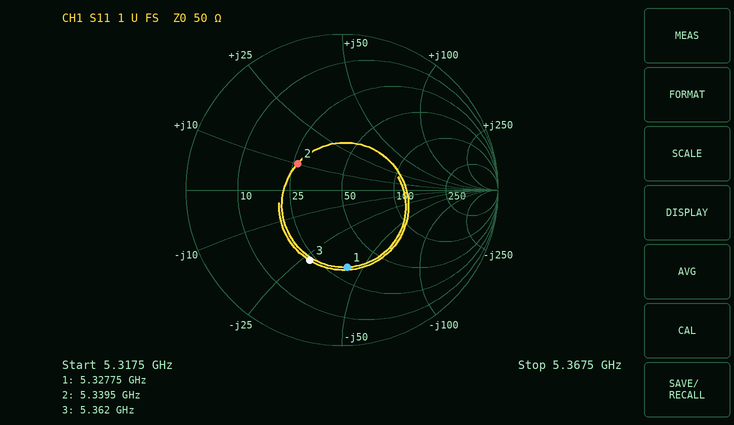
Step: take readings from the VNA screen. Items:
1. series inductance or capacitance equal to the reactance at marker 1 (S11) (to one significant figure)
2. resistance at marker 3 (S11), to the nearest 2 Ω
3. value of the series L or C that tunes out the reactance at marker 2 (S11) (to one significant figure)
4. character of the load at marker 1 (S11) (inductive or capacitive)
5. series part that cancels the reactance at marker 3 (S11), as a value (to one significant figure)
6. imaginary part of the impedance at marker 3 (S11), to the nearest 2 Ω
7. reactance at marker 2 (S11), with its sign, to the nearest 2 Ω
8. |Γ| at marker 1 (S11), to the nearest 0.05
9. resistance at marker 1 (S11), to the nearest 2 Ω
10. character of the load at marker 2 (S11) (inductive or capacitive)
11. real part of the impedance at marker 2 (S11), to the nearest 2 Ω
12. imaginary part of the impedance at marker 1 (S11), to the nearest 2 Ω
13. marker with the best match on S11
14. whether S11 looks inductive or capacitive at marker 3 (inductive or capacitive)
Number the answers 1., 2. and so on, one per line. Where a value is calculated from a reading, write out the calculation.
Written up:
1. C = 1/(2π × 5.32775 GHz × 42 Ω) ≈ 711 fF, so 700 fF to one significant figure
2. 22 Ω
3. C = 1/(2π × 5.3395 GHz × 10 Ω) ≈ 3 pF
4. capacitive
5. L = 28 Ω/(2π × 5.362 GHz) ≈ 831 pH, so 800 pH to one significant figure
6. -28 Ω
7. +10 Ω
8. 0.50
9. 32 Ω
10. inductive
11. 26 Ω
12. -42 Ω
13. marker 2
14. capacitive
